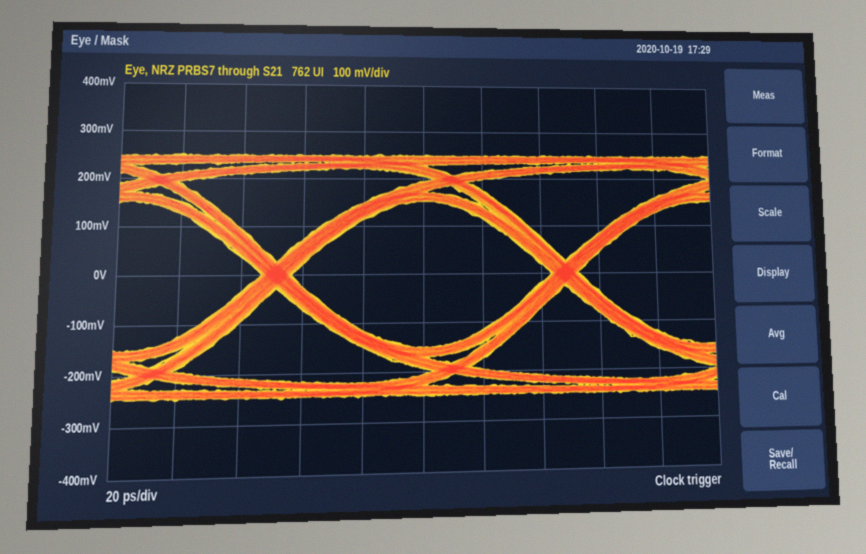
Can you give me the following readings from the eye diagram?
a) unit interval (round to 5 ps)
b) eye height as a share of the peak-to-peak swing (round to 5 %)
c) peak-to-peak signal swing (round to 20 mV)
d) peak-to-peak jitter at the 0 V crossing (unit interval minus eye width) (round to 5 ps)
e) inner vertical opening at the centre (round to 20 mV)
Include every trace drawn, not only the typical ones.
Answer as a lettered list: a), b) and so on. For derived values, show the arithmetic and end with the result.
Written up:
a) 95 ps
b) 300 mV / 500 mV ≈ 60 %
c) 500 mV
d) 10 ps
e) 300 mV
